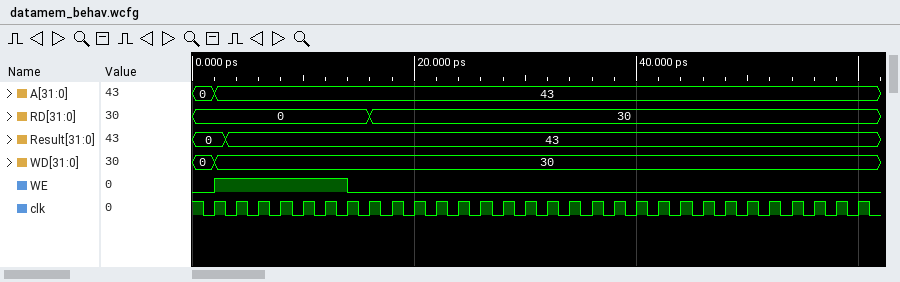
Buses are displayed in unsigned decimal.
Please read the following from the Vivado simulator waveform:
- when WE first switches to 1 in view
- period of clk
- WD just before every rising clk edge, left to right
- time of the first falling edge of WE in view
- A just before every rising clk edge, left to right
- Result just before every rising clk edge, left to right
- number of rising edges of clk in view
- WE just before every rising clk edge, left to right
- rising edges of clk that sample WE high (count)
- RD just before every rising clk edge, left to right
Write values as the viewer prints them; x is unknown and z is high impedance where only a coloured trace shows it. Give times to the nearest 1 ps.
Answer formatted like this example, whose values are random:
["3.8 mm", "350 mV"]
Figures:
["2 ps", "2 ps", "0, 30, 30, 30, 30, 30, 30, 30, 30, 30, 30, 30, 30, 30, 30, 30, 30, 30, 30, 30, 30, 30, 30, 30, 30, 30, 30, 30, 30, 30", "14 ps", "0, 43, 43, 43, 43, 43, 43, 43, 43, 43, 43, 43, 43, 43, 43, 43, 43, 43, 43, 43, 43, 43, 43, 43, 43, 43, 43, 43, 43, 43", "0, 43, 43, 43, 43, 43, 43, 43, 43, 43, 43, 43, 43, 43, 43, 43, 43, 43, 43, 43, 43, 43, 43, 43, 43, 43, 43, 43, 43, 43", "30", "0 1 1 1 1 1 1 0 0 0 0 0 0 0 0 0 0 0 0 0 0 0 0 0 0 0 0 0 0 0", "6", "0, 0, 0, 0, 0, 0, 0, 0, 30, 30, 30, 30, 30, 30, 30, 30, 30, 30, 30, 30, 30, 30, 30, 30, 30, 30, 30, 30, 30, 30"]
